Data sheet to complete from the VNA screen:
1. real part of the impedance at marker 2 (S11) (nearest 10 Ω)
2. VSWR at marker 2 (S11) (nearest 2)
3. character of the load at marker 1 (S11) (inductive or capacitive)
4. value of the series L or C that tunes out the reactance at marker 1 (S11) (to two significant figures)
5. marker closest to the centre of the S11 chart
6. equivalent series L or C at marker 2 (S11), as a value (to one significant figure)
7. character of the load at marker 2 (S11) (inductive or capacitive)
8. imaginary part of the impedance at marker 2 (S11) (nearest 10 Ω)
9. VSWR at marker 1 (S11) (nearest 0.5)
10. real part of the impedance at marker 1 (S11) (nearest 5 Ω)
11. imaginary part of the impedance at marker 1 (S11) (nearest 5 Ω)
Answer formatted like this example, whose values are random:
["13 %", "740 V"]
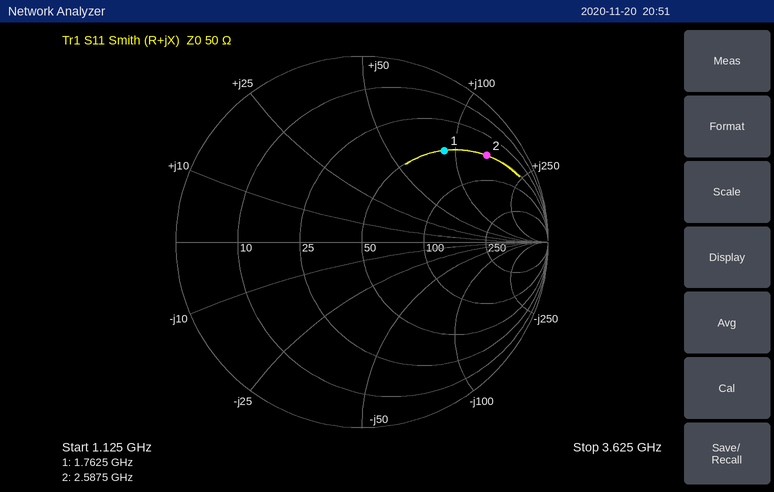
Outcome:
["50 Ω", "10", "inductive", "1.0 pF", "marker 1", "9 nH", "inductive", "+140 Ω", "5.0", "50 Ω", "+90 Ω"]
